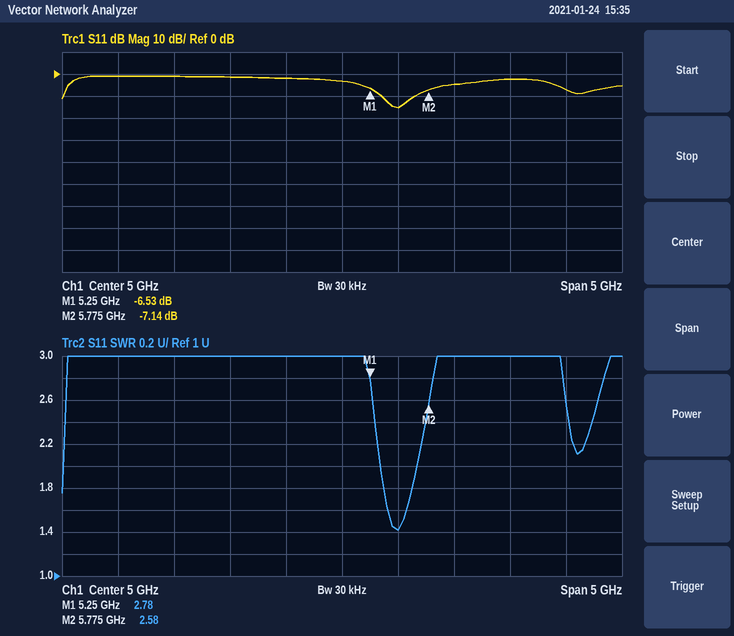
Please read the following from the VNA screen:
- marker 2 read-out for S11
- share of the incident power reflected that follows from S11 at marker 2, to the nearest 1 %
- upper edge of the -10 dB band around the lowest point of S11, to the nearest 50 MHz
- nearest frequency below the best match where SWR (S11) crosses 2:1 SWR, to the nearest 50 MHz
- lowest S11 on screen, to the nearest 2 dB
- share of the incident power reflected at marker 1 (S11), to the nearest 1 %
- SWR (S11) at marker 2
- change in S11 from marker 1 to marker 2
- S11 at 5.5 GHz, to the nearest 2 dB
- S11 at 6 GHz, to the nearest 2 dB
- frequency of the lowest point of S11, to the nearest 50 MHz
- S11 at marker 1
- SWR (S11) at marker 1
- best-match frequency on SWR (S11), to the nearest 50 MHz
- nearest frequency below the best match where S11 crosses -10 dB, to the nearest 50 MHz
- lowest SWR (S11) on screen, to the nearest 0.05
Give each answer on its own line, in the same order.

-7.14 dB
19 %
5.65 GHz
5.35 GHz
-16 dB
22 %
2.58
-0.61 dB
-16 dB
-4 dB
5.50 GHz
-6.53 dB
2.78
5.50 GHz
5.35 GHz
1.40
